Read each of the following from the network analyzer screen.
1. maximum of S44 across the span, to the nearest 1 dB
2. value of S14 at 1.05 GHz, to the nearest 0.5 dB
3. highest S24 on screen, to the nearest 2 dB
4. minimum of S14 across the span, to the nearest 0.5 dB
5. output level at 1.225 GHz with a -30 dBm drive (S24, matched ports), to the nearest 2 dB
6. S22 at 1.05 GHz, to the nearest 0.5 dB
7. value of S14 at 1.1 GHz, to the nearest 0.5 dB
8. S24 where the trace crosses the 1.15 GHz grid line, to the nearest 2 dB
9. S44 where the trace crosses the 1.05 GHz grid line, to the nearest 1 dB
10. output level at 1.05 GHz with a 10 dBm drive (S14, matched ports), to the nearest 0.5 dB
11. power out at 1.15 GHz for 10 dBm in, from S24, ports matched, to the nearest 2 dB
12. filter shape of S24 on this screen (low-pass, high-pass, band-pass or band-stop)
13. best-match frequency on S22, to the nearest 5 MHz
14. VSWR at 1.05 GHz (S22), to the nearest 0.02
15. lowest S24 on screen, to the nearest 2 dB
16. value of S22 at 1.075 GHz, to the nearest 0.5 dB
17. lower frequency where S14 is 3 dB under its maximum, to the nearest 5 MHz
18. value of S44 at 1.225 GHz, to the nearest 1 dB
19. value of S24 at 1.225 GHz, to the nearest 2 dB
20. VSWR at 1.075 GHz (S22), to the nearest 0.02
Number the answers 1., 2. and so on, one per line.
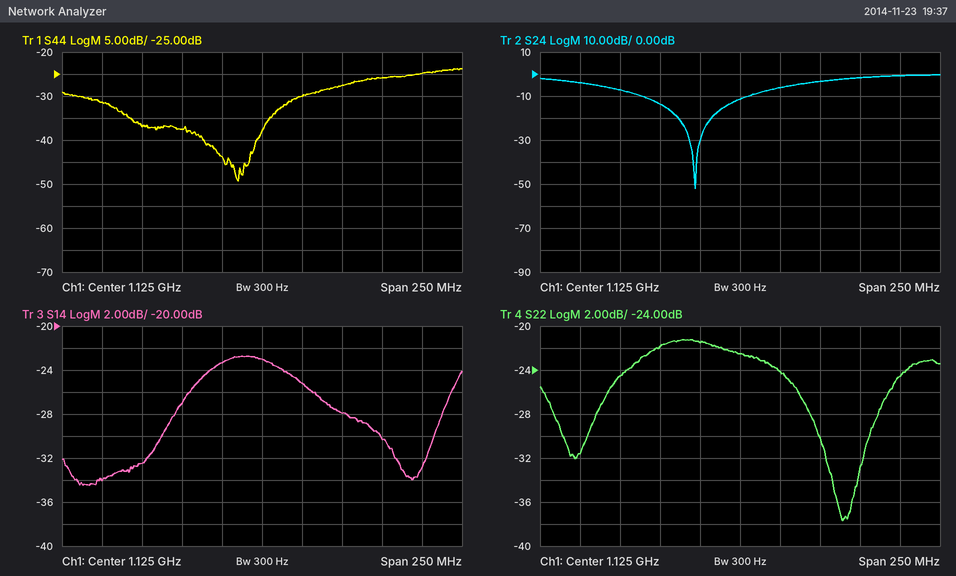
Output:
1. -24 dB
2. -32.5 dB
3. 0 dB
4. -34.5 dB
5. -30 dBm
6. -24.5 dB
7. -23.5 dB
8. -6 dB
9. -37 dB
10. -22.5 dBm
11. 4 dBm
12. band-stop
13. 1.190 GHz
14. 1.12
15. -52 dB
16. -22.0 dB
17. 1.080 GHz
18. -25 dB
19. 0 dB
20. 1.18
